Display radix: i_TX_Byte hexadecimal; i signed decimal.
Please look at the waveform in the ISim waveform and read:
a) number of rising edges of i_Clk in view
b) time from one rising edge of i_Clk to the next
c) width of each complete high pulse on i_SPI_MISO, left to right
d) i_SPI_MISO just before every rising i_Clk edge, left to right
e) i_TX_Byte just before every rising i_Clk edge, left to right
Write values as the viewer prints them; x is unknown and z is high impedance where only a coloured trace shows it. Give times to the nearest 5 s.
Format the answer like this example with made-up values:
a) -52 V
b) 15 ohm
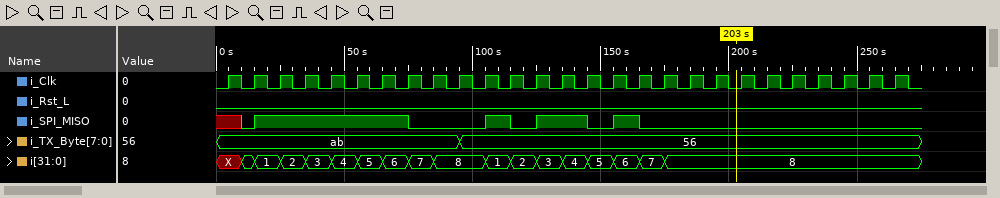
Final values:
a) 27
b) 10 s
c) 60 s, 10 s, 20 s, 10 s
d) x 0 1 1 1 1 1 1 0 0 0 1 0 1 1 0 1 0 0 0 0 0 0 0 0 0 0
e) ab, ab, ab, ab, ab, ab, ab, ab, ab, ab, 56, 56, 56, 56, 56, 56, 56, 56, 56, 56, 56, 56, 56, 56, 56, 56, 56
